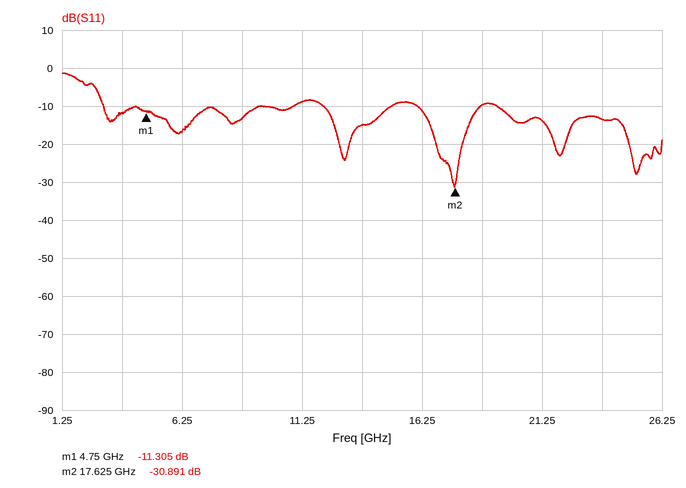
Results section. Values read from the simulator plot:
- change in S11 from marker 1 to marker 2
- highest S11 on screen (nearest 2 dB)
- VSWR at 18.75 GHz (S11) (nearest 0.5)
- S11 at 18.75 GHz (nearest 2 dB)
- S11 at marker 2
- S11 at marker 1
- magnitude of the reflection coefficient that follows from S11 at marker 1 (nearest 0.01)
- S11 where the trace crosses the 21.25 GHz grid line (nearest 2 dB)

-19.586 dB
-2 dB
2.0
-10 dB
-30.891 dB
-11.305 dB
0.27
-14 dB
